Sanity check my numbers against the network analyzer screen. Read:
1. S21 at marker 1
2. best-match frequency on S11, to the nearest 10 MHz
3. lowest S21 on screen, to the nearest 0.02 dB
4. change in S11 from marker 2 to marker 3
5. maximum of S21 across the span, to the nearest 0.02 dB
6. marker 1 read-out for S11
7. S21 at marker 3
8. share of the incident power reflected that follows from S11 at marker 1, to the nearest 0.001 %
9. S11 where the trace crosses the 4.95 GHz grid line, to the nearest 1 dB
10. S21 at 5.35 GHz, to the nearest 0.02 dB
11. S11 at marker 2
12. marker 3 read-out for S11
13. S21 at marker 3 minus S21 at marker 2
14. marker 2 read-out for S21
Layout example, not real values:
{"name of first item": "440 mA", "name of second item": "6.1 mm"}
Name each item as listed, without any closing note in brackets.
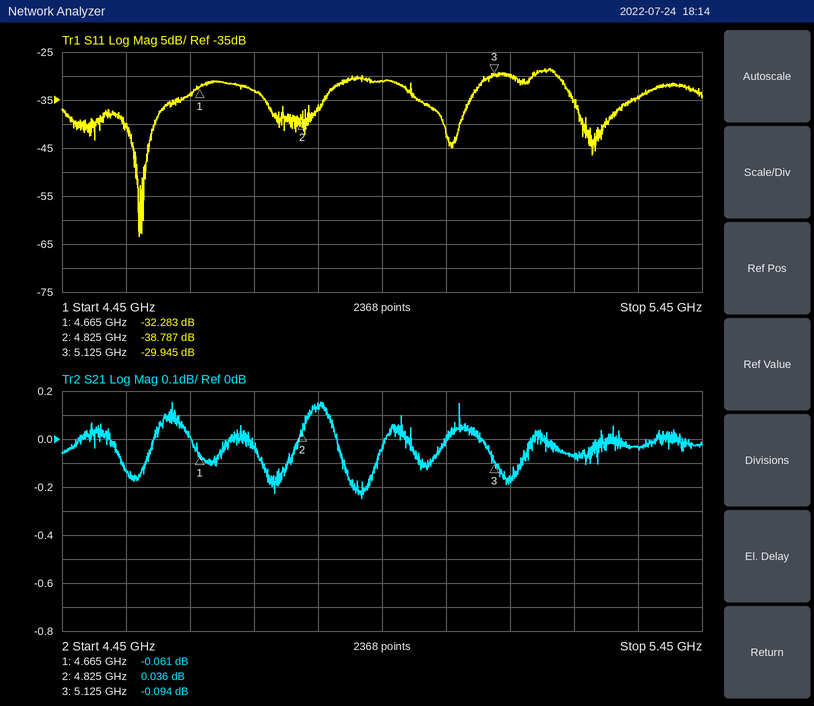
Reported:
{"S21 at marker 1": "-0.061 dB", "best-match frequency on S11, to the nearest 10 MHz": "4.57 GHz", "lowest S21 on screen, to the nearest 0.02 dB": "-0.24 dB", "change in S11 from marker 2 to marker 3": "8.842 dB", "maximum of S21 across the span, to the nearest 0.02 dB": "0.16 dB", "marker 1 read-out for S11": "-32.283 dB", "S21 at marker 3": "-0.094 dB", "share of the incident power reflected that follows from S11 at marker 1, to the nearest 0.001 %": "0.059 %", "S11 where the trace crosses the 4.95 GHz grid line, to the nearest 1 dB": "-31 dB", "S21 at 5.35 GHz, to the nearest 0.02 dB": "-0.04 dB", "S11 at marker 2": "-38.787 dB", "marker 3 read-out for S11": "-29.945 dB", "S21 at marker 3 minus S21 at marker 2": "-0.130 dB", "marker 2 read-out for S21": "0.036 dB"}
